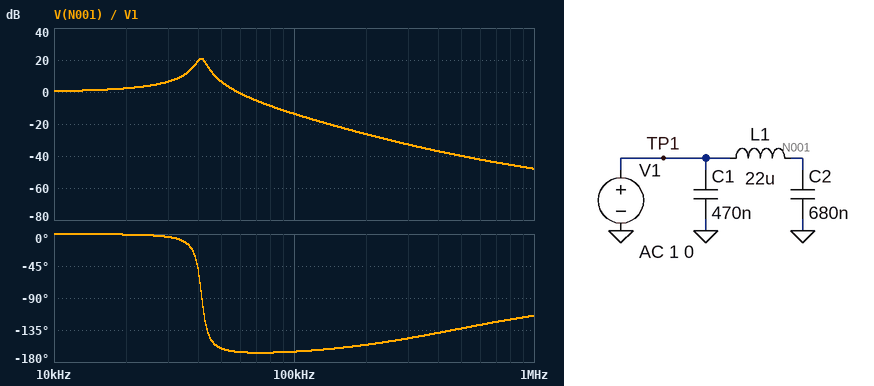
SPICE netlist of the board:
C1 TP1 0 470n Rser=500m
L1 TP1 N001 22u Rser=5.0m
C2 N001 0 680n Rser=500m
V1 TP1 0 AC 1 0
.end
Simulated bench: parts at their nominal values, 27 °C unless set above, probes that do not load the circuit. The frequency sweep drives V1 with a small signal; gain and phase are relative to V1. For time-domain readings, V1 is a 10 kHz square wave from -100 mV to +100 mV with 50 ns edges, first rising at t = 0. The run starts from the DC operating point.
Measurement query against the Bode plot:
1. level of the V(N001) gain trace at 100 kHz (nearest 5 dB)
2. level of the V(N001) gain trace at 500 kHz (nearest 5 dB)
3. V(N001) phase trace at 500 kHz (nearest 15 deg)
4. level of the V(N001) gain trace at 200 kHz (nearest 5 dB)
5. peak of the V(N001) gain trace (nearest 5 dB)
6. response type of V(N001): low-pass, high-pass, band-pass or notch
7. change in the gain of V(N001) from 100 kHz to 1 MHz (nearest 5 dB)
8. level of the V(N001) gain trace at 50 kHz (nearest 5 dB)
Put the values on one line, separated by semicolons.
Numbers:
-15 dB; -40 dB; -135 deg; -25 dB; 20 dB; low-pass; -35 dB; 5 dB
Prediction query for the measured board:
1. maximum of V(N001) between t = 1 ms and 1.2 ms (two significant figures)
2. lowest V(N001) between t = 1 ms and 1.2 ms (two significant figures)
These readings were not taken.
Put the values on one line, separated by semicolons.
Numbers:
210 mV; -210 mV
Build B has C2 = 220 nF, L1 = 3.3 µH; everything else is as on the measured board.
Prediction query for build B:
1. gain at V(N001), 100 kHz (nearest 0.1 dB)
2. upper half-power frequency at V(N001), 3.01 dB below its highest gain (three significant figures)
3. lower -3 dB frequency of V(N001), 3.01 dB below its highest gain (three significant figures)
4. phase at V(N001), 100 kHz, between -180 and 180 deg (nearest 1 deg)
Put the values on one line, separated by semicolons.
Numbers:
2.9 dB; 198 kHz; 173 kHz; -2 deg
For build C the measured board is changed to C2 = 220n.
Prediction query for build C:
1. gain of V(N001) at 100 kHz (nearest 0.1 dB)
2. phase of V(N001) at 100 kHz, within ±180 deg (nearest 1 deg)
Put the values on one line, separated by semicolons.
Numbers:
0.8 dB; -172 deg
